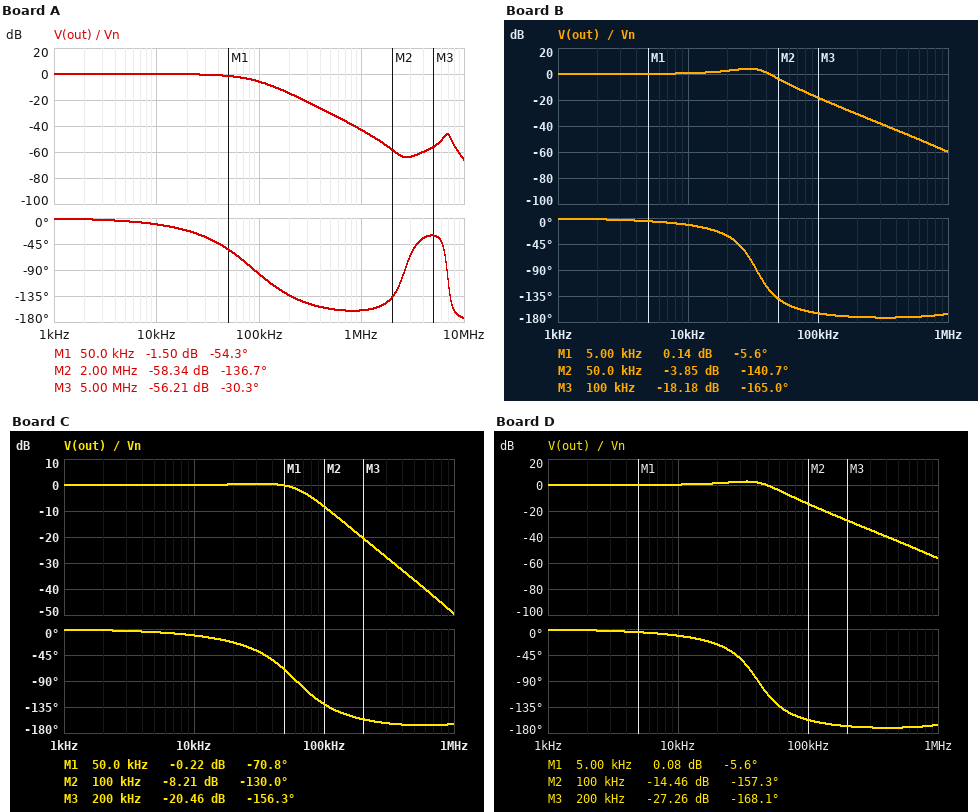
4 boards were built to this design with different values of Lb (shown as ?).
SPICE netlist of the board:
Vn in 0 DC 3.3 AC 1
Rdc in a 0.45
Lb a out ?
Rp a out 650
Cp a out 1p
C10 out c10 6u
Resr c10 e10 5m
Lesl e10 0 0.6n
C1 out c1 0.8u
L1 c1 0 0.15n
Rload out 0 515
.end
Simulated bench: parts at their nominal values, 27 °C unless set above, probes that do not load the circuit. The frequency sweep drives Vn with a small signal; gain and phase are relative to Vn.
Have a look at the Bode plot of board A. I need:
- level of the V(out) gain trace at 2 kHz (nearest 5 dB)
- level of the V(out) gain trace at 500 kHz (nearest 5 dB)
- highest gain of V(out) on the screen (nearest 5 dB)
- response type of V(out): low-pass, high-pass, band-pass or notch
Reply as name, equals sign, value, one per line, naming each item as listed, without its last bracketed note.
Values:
level of the V(out) gain trace at 2 kHz = 0 dB
level of the V(out) gain trace at 500 kHz = -30 dB
highest gain of V(out) on the screen = 0 dB
response type of V(out): low-pass, high-pass, band-pass or notch = low-pass
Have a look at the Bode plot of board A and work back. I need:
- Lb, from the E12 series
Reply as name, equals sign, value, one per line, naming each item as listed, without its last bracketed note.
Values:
Lb, from the E12 series = 470 nH
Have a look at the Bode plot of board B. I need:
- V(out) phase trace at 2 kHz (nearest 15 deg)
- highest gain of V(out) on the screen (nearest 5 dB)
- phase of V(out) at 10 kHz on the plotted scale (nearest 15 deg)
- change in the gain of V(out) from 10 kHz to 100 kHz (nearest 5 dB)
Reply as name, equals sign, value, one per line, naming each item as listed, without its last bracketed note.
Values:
V(out) phase trace at 2 kHz = 0 deg
highest gain of V(out) on the screen = 5 dB
phase of V(out) at 10 kHz on the plotted scale = -15 deg
change in the gain of V(out) from 10 kHz to 100 kHz = -20 dB
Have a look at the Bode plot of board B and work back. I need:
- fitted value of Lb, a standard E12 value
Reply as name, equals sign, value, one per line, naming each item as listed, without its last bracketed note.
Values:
fitted value of Lb, a standard E12 value = 3.3 µH
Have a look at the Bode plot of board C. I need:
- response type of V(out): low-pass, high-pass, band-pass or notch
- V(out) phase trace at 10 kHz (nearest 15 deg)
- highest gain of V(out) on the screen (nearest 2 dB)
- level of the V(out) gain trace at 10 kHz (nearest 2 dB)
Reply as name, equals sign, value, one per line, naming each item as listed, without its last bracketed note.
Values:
response type of V(out): low-pass, high-pass, band-pass or notch = low-pass
V(out) phase trace at 10 kHz = -15 deg
highest gain of V(out) on the screen = 0 dB
level of the V(out) gain trace at 10 kHz = 0 dB
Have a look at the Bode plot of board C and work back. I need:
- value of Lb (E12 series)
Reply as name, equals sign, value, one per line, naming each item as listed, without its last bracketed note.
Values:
value of Lb = 1 µH
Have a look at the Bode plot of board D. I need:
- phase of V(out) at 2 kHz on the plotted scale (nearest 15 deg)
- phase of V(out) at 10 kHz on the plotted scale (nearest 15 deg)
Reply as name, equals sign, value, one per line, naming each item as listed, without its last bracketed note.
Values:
phase of V(out) at 2 kHz on the plotted scale = 0 deg
phase of V(out) at 10 kHz on the plotted scale = -15 deg
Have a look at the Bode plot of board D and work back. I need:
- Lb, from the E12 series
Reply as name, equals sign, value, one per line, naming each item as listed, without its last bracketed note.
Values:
Lb, from the E12 series = 2.2 µH
